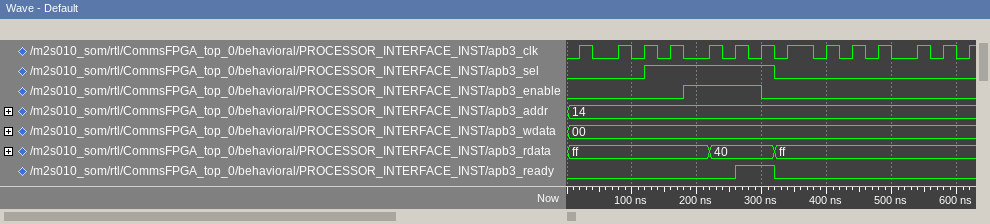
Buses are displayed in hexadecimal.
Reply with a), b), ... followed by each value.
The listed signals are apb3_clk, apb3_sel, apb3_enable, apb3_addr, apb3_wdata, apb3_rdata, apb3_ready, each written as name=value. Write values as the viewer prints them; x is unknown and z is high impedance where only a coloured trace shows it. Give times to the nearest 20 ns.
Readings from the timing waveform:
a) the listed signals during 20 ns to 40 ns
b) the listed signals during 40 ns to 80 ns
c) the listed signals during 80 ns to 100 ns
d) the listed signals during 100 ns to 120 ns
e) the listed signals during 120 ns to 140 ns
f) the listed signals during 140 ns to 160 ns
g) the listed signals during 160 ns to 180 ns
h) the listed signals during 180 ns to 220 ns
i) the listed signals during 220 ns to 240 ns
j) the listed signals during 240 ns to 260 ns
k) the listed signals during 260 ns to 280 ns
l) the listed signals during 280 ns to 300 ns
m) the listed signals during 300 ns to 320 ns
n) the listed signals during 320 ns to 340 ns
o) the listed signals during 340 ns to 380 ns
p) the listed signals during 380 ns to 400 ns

a) apb3_clk=1, apb3_sel=0, apb3_enable=0, apb3_addr=14, apb3_wdata=00, apb3_rdata=ff, apb3_ready=0
b) apb3_clk=0, apb3_sel=0, apb3_enable=0, apb3_addr=14, apb3_wdata=00, apb3_rdata=ff, apb3_ready=0
c) apb3_clk=1, apb3_sel=0, apb3_enable=0, apb3_addr=14, apb3_wdata=00, apb3_rdata=ff, apb3_ready=0
d) apb3_clk=0, apb3_sel=0, apb3_enable=0, apb3_addr=14, apb3_wdata=00, apb3_rdata=ff, apb3_ready=0
e) apb3_clk=1, apb3_sel=1, apb3_enable=0, apb3_addr=14, apb3_wdata=00, apb3_rdata=ff, apb3_ready=0
f) apb3_clk=0, apb3_sel=1, apb3_enable=0, apb3_addr=14, apb3_wdata=00, apb3_rdata=ff, apb3_ready=0
g) apb3_clk=1, apb3_sel=1, apb3_enable=0, apb3_addr=14, apb3_wdata=00, apb3_rdata=ff, apb3_ready=0
h) apb3_clk=0, apb3_sel=1, apb3_enable=1, apb3_addr=14, apb3_wdata=00, apb3_rdata=ff, apb3_ready=0
i) apb3_clk=1, apb3_sel=1, apb3_enable=1, apb3_addr=14, apb3_wdata=00, apb3_rdata=40, apb3_ready=0
j) apb3_clk=0, apb3_sel=1, apb3_enable=1, apb3_addr=14, apb3_wdata=00, apb3_rdata=40, apb3_ready=0
k) apb3_clk=1, apb3_sel=1, apb3_enable=1, apb3_addr=14, apb3_wdata=00, apb3_rdata=40, apb3_ready=1
l) apb3_clk=0, apb3_sel=1, apb3_enable=1, apb3_addr=14, apb3_wdata=00, apb3_rdata=40, apb3_ready=1
m) apb3_clk=1, apb3_sel=1, apb3_enable=0, apb3_addr=14, apb3_wdata=00, apb3_rdata=40, apb3_ready=1
n) apb3_clk=0, apb3_sel=0, apb3_enable=0, apb3_addr=14, apb3_wdata=00, apb3_rdata=ff, apb3_ready=0
o) apb3_clk=1, apb3_sel=0, apb3_enable=0, apb3_addr=14, apb3_wdata=00, apb3_rdata=ff, apb3_ready=0
p) apb3_clk=0, apb3_sel=0, apb3_enable=0, apb3_addr=14, apb3_wdata=00, apb3_rdata=ff, apb3_ready=0
